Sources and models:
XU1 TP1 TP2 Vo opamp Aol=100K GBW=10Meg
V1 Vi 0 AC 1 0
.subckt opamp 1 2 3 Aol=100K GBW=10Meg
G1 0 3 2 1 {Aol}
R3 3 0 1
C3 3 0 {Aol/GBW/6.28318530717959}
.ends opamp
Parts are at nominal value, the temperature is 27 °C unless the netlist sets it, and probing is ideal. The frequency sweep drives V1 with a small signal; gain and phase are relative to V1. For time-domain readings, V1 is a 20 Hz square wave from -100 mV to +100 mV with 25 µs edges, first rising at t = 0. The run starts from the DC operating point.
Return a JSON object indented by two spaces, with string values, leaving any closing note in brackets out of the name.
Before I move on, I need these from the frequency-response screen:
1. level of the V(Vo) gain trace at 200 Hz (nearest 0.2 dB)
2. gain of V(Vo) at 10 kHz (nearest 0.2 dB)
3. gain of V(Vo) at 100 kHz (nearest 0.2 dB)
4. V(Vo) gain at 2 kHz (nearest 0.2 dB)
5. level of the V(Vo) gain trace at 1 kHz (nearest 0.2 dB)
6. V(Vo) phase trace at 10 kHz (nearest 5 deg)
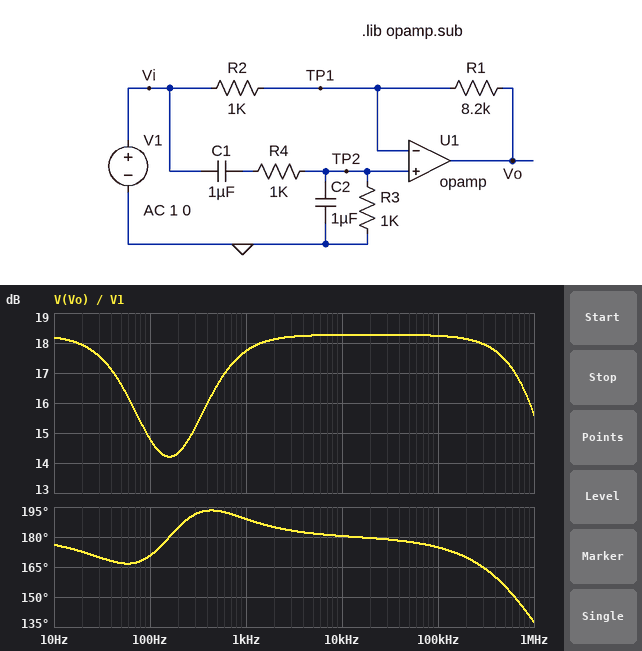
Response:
{
  "level of the V(Vo) gain trace at 200 Hz": "14.4 dB",
  "gain of V(Vo) at 10 kHz": "18.2 dB",
  "gain of V(Vo) at 100 kHz": "18.2 dB",
  "V(Vo) gain at 2 kHz": "18.2 dB",
  "level of the V(Vo) gain trace at 1 kHz": "17.8 dB",
  "V(Vo) phase trace at 10 kHz": "180 deg"
}
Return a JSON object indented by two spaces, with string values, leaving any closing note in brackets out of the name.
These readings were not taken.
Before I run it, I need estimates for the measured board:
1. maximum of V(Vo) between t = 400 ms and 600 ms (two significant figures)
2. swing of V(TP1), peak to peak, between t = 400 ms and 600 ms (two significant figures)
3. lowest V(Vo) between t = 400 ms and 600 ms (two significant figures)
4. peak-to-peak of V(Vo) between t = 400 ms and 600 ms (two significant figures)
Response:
{
  "maximum of V(Vo) between t = 400 ms and 600 ms": "820 mV",
  "swing of V(TP1), peak to peak, between t = 400 ms and 600 ms": "110 mV",
  "lowest V(Vo) between t = 400 ms and 600 ms": "-820 mV",
  "peak-to-peak of V(Vo) between t = 400 ms and 600 ms": "1.6 V"
}
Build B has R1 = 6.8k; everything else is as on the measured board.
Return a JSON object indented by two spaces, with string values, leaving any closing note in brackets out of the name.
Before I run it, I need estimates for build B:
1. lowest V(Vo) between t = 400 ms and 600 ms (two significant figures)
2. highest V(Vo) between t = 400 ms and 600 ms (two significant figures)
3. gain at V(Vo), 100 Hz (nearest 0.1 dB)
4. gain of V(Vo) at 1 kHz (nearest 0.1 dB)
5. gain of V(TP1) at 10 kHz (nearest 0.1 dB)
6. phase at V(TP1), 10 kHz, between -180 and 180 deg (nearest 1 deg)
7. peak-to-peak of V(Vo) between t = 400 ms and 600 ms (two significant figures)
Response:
{
  "lowest V(Vo) between t = 400 ms and 600 ms": "-680 mV",
  "highest V(Vo) between t = 400 ms and 600 ms": "680 mV",
  "gain at V(Vo), 100 Hz": "13.1 dB",
  "gain of V(Vo) at 1 kHz": "16.1 dB",
  "gain of V(TP1) at 10 kHz": "-40.8 dB",
  "phase at V(TP1), 10 kHz, between -180 and 180 deg": "-85 deg",
  "peak-to-peak of V(Vo) between t = 400 ms and 600 ms": "1.4 V"
}
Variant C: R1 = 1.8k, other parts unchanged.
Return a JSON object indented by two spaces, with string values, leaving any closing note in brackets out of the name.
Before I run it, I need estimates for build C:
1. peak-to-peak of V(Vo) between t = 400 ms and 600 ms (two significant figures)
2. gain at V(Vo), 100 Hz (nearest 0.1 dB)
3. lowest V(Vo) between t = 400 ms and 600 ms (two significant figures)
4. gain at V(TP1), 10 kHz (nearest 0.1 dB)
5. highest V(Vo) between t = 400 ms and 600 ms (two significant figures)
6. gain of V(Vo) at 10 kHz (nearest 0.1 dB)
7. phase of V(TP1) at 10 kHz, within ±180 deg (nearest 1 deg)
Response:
{
  "peak-to-peak of V(Vo) between t = 400 ms and 600 ms": "360 mV",
  "gain at V(Vo), 100 Hz": "-0.1 dB",
  "lowest V(Vo) between t = 400 ms and 600 ms": "-180 mV",
  "gain at V(TP1), 10 kHz": "-37.0 dB",
  "highest V(Vo) between t = 400 ms and 600 ms": "180 mV",
  "gain of V(Vo) at 10 kHz": "5.1 dB",
  "phase of V(TP1) at 10 kHz, within ±180 deg": "-87 deg"
}
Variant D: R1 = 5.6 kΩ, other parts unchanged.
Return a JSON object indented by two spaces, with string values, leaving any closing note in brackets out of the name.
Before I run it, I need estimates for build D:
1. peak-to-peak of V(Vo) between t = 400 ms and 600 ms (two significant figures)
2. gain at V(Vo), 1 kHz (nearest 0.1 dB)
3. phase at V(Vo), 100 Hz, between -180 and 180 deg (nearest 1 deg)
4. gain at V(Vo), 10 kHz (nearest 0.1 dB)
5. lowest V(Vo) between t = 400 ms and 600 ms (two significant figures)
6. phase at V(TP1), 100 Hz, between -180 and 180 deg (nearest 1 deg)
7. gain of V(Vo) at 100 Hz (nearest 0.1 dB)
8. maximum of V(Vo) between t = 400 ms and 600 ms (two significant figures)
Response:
{
  "peak-to-peak of V(Vo) between t = 400 ms and 600 ms": "1.1 V",
  "gain at V(Vo), 1 kHz": "14.4 dB",
  "phase at V(Vo), 100 Hz, between -180 and 180 deg": "170 deg",
  "gain at V(Vo), 10 kHz": "15.0 dB",
  "lowest V(Vo) between t = 400 ms and 600 ms": "-560 mV",
  "phase at V(TP1), 100 Hz, between -180 and 180 deg": "18 deg",
  "gain of V(Vo) at 100 Hz": "11.3 dB",
  "maximum of V(Vo) between t = 400 ms and 600 ms": "560 mV"
}
